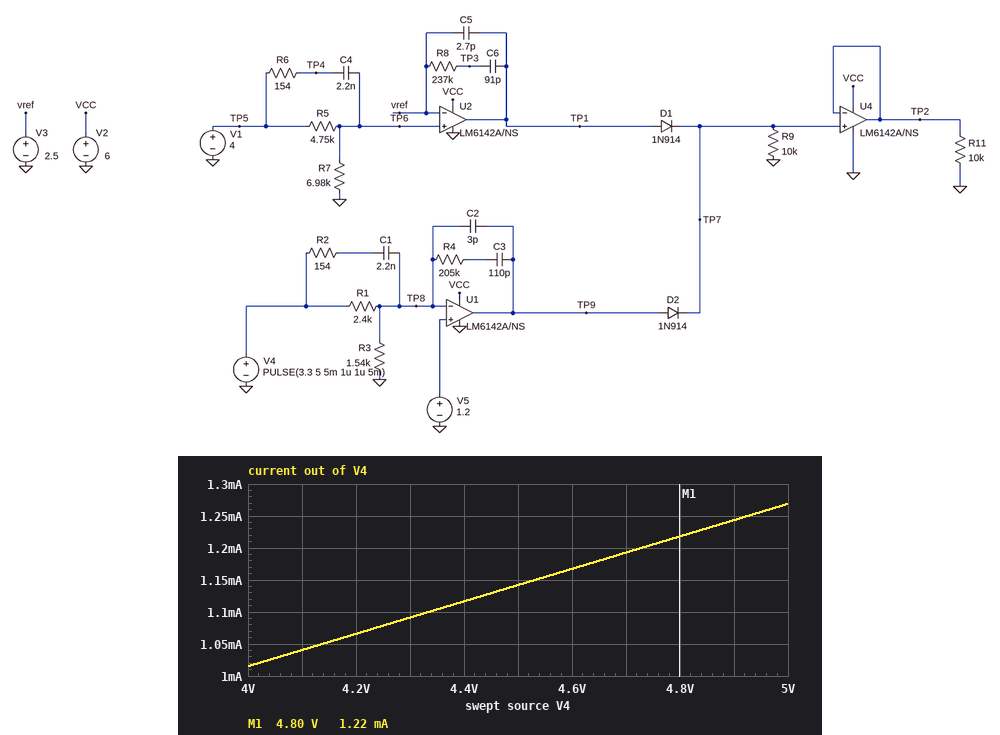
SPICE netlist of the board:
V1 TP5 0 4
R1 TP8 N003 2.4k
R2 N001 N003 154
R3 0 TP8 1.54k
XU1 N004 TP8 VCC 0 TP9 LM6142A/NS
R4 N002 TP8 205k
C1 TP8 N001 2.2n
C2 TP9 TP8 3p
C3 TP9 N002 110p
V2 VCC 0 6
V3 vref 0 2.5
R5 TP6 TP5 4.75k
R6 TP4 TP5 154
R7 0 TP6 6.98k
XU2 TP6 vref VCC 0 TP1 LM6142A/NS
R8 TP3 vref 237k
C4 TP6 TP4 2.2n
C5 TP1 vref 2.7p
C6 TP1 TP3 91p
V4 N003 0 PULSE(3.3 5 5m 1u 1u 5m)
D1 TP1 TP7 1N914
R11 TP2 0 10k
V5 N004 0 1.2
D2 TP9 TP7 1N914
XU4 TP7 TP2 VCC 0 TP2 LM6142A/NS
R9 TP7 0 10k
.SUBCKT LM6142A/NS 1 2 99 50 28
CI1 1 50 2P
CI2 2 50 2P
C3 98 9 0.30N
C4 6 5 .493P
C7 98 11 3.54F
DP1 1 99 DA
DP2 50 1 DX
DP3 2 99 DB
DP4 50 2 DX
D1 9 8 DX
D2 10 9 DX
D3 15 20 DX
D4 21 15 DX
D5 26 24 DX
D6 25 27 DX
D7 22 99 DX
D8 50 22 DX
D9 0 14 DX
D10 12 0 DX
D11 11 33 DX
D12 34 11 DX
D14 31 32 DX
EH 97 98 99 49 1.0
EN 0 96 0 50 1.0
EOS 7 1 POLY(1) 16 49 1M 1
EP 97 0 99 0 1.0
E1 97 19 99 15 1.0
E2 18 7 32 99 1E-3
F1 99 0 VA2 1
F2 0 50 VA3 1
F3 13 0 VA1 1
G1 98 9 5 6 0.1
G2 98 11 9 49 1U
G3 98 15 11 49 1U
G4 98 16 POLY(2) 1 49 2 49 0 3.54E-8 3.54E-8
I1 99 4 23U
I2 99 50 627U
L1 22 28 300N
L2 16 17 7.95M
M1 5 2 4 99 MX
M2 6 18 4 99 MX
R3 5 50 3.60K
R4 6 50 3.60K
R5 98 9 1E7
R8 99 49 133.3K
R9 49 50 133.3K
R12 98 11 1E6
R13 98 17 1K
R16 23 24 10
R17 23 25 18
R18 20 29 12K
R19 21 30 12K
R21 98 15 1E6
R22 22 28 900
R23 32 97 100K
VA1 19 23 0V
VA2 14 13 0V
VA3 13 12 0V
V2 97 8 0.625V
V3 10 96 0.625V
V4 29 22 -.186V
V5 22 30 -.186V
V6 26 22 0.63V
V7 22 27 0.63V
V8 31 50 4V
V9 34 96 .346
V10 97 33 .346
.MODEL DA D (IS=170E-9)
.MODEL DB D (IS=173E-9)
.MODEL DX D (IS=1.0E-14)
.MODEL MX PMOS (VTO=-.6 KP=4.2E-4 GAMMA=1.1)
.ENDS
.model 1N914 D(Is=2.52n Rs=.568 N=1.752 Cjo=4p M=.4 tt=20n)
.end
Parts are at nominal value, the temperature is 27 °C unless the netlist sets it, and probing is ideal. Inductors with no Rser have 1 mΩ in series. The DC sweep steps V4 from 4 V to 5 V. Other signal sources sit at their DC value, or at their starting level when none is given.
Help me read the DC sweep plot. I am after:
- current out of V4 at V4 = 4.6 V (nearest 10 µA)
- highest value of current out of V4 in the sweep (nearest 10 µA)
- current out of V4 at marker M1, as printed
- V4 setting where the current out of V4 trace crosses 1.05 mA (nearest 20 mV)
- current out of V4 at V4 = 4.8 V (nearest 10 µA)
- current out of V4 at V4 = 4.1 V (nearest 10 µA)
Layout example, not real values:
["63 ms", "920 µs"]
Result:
["1.17 mA", "1.27 mA", "1.22 mA", "4.14 V", "1.22 mA", "1.04 mA"]
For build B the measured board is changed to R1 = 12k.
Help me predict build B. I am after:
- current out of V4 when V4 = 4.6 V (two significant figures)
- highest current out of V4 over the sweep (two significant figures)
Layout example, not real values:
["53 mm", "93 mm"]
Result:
["340 µA", "370 µA"]
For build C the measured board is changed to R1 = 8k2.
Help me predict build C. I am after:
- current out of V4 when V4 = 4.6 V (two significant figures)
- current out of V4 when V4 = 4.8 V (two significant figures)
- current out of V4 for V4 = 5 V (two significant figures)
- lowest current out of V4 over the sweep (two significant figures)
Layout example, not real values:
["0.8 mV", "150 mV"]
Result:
["470 µA", "490 µA", "510 µA", "410 µA"]
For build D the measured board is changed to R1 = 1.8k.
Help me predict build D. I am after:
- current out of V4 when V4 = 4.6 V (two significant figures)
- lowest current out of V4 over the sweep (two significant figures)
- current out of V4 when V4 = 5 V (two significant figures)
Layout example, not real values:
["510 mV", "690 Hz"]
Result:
["1.4 mA", "1.2 mA", "1.5 mA"]
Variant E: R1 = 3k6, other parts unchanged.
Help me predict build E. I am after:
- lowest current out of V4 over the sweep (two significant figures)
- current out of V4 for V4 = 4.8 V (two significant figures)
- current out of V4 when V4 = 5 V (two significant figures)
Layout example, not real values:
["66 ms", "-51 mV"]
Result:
["780 µA", "930 µA", "970 µA"]
